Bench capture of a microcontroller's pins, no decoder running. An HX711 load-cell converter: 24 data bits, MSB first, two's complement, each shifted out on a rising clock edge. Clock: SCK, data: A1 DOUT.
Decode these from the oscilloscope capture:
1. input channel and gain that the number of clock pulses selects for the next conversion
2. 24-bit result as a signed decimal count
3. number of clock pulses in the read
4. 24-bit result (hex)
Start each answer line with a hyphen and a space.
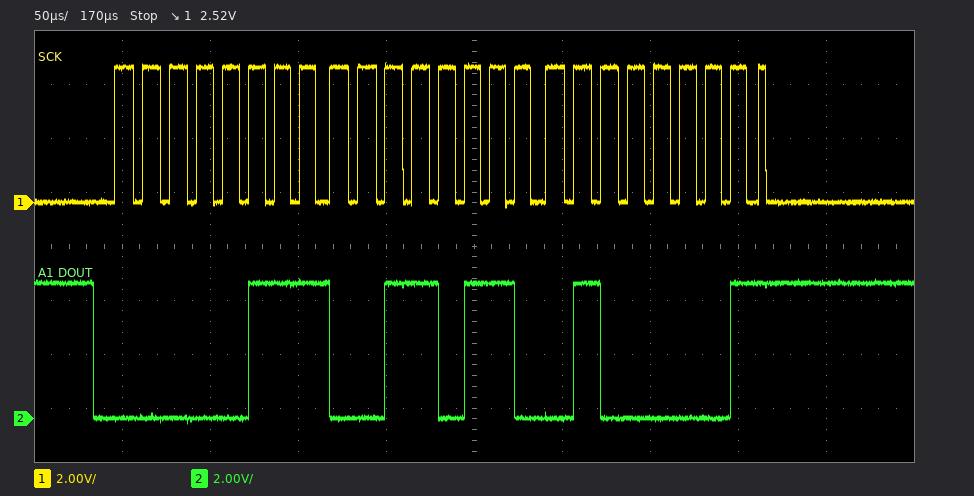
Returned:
- channel A, gain 128
- 472641
- 25
- 0x073641
